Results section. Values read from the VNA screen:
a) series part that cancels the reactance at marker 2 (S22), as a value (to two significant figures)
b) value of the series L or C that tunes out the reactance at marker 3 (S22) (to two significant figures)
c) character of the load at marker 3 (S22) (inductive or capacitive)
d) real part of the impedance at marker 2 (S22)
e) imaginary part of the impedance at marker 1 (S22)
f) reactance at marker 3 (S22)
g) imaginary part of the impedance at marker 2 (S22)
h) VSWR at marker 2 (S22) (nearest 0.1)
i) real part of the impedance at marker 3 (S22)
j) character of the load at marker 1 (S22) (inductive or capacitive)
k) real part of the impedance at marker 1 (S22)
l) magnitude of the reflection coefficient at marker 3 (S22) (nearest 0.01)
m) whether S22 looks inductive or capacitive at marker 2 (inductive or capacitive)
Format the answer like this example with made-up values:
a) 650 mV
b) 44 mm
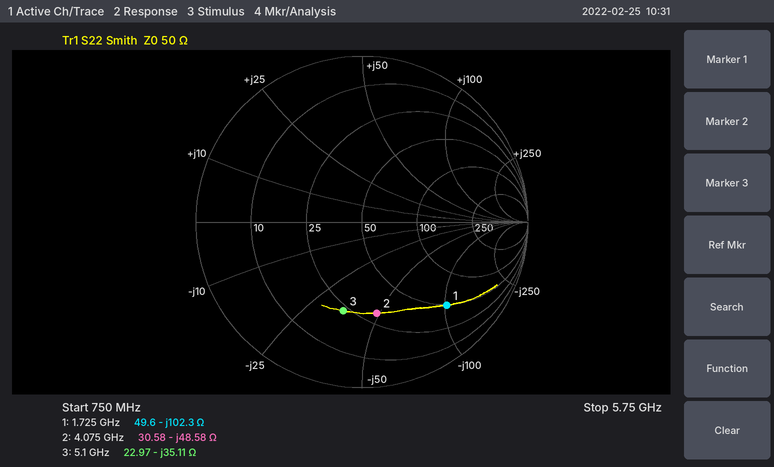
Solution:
a) 1.9 nH
b) 1.1 nH
c) capacitive
d) 30.58 Ω
e) -102.3 Ω
f) -35.11 Ω
g) -48.58 Ω
h) 3.5
i) 22.97 Ω
j) capacitive
k) 49.6 Ω
l) 0.55
m) capacitive
